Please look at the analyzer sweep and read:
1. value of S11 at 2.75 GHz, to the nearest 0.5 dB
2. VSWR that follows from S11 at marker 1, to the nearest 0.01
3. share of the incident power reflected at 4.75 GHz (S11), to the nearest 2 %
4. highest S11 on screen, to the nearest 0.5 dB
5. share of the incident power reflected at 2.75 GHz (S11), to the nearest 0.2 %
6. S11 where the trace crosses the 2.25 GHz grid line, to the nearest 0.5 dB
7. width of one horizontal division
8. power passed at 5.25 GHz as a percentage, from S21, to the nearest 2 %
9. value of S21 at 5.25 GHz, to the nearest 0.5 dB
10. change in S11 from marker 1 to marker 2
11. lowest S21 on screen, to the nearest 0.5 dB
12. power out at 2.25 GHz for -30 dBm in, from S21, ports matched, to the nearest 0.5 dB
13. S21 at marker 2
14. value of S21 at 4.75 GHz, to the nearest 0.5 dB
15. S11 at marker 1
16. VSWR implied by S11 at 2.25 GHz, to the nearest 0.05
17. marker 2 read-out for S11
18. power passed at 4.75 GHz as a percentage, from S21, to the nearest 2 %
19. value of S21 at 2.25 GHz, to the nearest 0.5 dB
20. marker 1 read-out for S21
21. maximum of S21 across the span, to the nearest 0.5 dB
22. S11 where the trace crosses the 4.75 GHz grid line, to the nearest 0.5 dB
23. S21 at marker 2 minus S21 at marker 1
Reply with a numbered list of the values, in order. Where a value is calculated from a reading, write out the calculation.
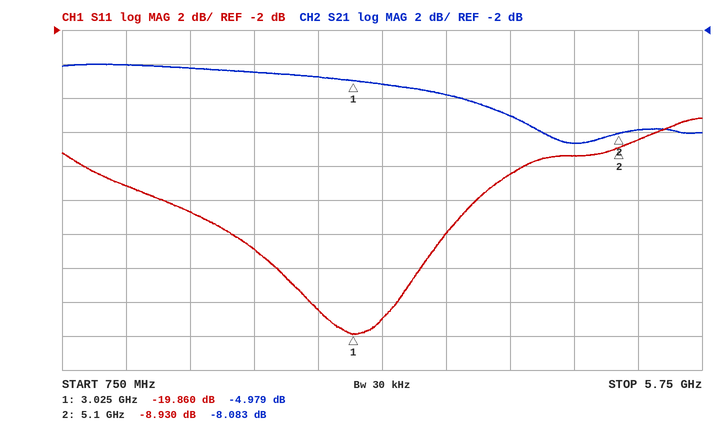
1. -18.5 dB
2. (1 + 0.1016)/(1 − 0.1016) ≈ 1.23
3. 10^(-9.5/10) ≈ 11.2 %, so 12 % to the nearest 2 %
4. -7.0 dB
5. 10^(-18.5/10) ≈ 1.4 %
6. -15.0 dB
7. 500 MHz
8. 10^(-8/10) ≈ 16 %
9. -8.0 dB
10. -8.93 − (-19.86) = 10.930 dB
11. -8.5 dB
12. -30 dBm + (-4.5 dB) = -34.5 dBm
13. -8.083 dB
14. -8.5 dB
15. -19.860 dB
16. |Γ| = 10^(-15/20) = 0.1778; VSWR = (1 + 0.1778)/(1 − 0.1778) ≈ 1.43, so 1.45 to the nearest 0.05
17. -8.930 dB
18. 10^(-8.5/10) ≈ 14 %
19. -4.5 dB
20. -4.979 dB
21. -4.0 dB
22. -9.5 dB
23. -8.083 − (-4.979) = -3.104 dB
